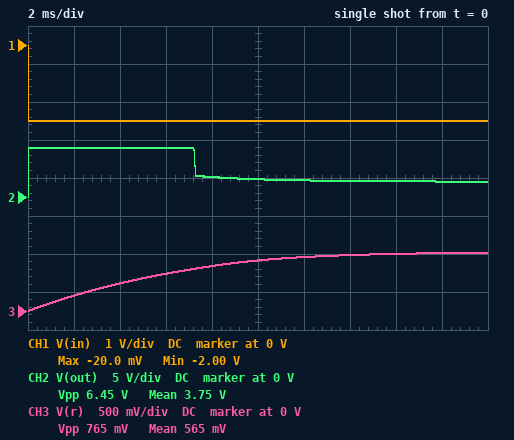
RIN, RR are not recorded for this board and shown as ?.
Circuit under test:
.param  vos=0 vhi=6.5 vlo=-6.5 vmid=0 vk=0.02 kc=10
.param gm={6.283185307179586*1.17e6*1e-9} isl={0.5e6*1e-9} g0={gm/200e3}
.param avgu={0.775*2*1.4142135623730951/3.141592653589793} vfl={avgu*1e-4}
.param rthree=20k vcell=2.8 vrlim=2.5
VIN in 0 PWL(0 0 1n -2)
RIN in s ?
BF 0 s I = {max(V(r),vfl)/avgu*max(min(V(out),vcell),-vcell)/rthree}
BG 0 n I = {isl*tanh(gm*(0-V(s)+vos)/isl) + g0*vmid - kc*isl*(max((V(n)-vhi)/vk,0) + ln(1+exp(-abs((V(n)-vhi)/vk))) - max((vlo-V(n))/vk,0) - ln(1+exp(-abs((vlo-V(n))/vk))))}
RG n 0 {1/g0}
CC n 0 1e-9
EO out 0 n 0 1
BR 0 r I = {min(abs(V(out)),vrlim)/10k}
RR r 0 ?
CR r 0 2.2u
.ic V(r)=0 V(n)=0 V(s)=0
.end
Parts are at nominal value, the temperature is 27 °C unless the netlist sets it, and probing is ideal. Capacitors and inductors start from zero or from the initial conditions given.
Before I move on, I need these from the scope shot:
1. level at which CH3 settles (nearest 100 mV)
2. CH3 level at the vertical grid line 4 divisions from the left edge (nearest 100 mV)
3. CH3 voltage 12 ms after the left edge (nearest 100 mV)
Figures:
800 mV
600 mV
700 mV
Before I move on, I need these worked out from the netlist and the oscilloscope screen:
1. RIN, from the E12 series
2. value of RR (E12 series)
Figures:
18 kΩ
3.9 kΩ
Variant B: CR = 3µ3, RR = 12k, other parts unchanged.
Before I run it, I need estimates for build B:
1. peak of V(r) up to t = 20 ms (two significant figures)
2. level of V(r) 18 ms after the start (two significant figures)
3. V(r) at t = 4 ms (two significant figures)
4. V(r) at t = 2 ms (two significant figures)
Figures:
1.0 V
960 mV
290 mV
150 mV
